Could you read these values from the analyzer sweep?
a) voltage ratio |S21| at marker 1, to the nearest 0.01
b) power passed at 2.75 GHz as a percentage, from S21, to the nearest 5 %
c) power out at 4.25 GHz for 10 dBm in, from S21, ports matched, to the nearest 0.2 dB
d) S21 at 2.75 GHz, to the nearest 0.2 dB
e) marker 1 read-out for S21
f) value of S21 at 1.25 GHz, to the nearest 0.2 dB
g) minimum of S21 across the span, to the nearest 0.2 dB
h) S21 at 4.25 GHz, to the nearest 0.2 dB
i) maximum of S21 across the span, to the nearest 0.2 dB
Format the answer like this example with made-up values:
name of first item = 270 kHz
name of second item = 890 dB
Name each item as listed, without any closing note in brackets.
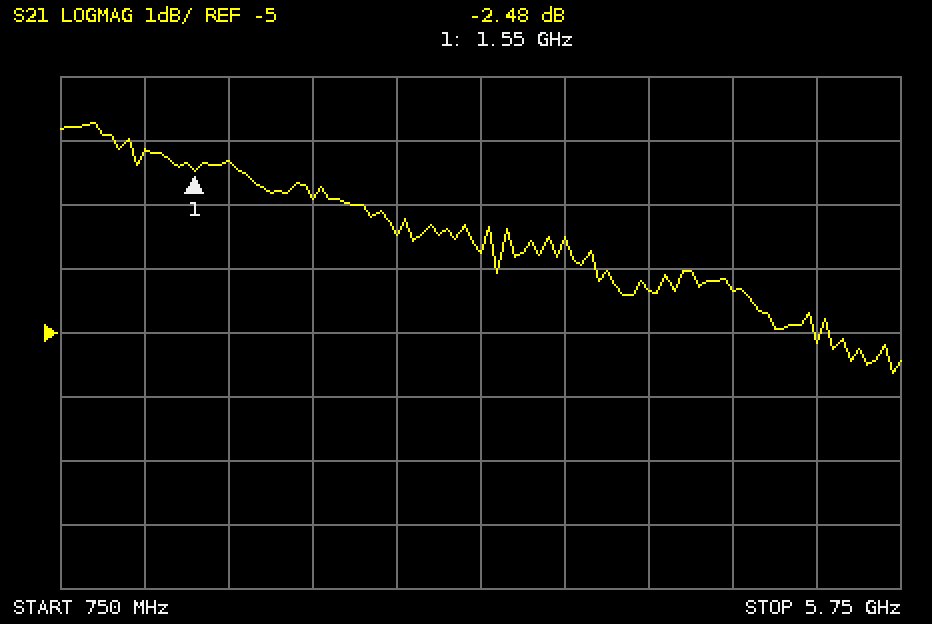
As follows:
voltage ratio |S21| at marker 1, to the nearest 0.01 = 0.75
power passed at 2.75 GHz as a percentage, from S21, to the nearest 5 % = 45 %
power out at 4.25 GHz for 10 dBm in, from S21, ports matched, to the nearest 0.2 dB = 5.6 dBm
S21 at 2.75 GHz, to the nearest 0.2 dB = -3.4 dB
marker 1 read-out for S21 = -2.48 dB
value of S21 at 1.25 GHz, to the nearest 0.2 dB = -2.2 dB
minimum of S21 across the span, to the nearest 0.2 dB = -5.6 dB
S21 at 4.25 GHz, to the nearest 0.2 dB = -4.4 dB
maximum of S21 across the span, to the nearest 0.2 dB = -1.8 dB
